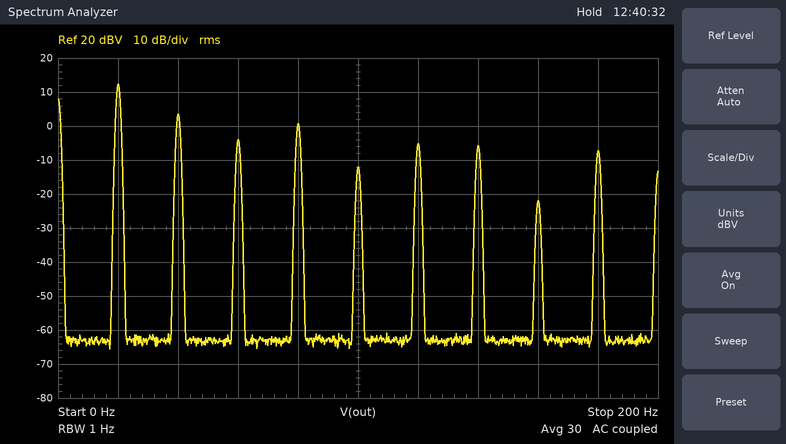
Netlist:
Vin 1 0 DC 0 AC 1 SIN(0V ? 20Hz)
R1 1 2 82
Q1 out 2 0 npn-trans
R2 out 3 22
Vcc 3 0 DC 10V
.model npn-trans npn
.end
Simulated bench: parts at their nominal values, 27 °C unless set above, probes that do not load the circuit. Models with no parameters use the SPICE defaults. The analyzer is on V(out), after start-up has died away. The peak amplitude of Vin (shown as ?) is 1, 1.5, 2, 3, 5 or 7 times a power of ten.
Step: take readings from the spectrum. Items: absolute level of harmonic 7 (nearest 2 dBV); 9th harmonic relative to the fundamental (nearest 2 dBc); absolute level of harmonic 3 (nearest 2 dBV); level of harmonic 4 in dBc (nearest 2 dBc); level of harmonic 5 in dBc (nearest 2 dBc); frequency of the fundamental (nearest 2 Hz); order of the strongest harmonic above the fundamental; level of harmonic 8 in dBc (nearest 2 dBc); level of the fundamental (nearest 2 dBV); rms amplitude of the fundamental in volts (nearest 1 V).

-6 dBV
-20 dBc
-4 dBV
-12 dBc
-24 dBc
20 Hz
2
-34 dBc
12 dBV
4 V
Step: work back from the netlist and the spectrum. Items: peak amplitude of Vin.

3 V
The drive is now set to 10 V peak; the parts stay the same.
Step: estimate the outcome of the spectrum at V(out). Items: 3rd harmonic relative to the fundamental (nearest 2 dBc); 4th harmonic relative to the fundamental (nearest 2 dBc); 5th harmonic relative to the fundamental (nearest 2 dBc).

-10 dBc
-20 dBc
-16 dBc
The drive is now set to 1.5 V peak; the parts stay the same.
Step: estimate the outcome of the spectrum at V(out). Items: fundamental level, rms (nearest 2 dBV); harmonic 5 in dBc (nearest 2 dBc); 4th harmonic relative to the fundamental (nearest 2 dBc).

10 dBV
-18 dBc
-26 dBc
